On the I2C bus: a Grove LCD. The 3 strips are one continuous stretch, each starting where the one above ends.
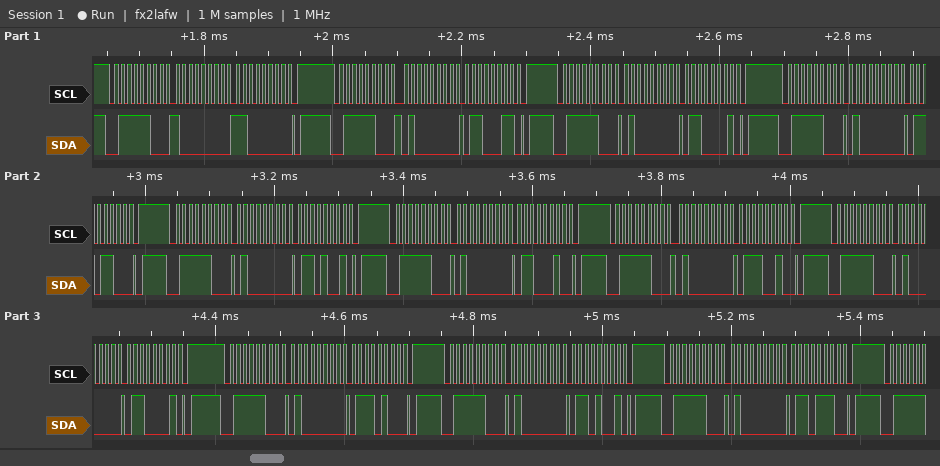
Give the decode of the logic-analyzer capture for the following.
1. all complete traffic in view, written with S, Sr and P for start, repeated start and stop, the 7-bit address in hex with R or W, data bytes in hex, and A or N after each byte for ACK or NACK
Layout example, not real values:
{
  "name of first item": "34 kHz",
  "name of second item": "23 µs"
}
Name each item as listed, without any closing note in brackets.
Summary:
{
  "all complete traffic in view, written with S, Sr and P for start, repeated start and stop, the 7-bit address in hex with R or W, data bytes in hex, and A or N after each byte for ACK or NACK": "S 3EW A 80 A C0 A P S 3EW A 40 A 63 A P S 3EW A 40 A 61 A P S 3EW A 40 A 6C A P S 3EW A 40 A 69 A P S 3EW A 40 A 62 A P S 3EW A 40 A 72 A P S 3EW A 40 A 61 A P S 3EW A 40 A 74 A P S 3EW A 40 A 69 A P S 3EW A 40 A 6E A P"
}
